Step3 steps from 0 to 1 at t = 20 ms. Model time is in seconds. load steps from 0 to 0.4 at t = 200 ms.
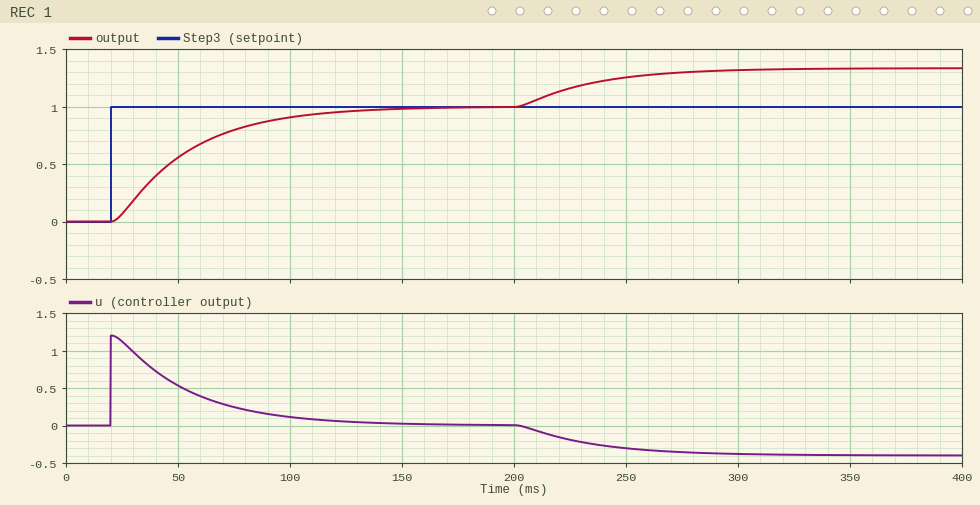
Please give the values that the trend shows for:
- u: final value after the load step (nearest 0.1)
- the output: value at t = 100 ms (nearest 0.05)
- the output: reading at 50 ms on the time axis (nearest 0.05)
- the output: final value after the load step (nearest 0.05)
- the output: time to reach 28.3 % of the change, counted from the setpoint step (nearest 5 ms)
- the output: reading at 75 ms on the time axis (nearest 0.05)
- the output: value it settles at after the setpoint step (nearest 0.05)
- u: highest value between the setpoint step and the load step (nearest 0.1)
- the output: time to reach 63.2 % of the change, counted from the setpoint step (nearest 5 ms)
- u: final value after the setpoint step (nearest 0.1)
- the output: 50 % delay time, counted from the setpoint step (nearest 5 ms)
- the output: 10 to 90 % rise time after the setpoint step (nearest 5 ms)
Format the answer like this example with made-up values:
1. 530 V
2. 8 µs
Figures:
1. -0.4
2. 0.90
3. 0.55
4. 1.35
5. 15 ms
6. 0.80
7. 1.00
8. 1.2
9. 35 ms
10. 0.0
11. 25 ms
12. 70 ms
